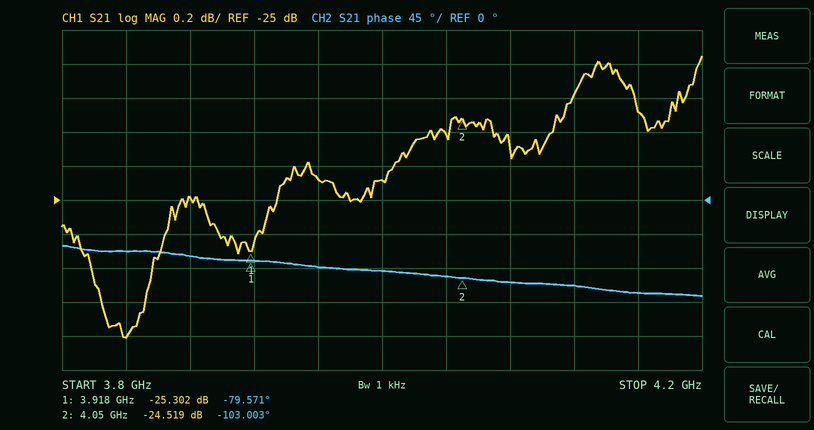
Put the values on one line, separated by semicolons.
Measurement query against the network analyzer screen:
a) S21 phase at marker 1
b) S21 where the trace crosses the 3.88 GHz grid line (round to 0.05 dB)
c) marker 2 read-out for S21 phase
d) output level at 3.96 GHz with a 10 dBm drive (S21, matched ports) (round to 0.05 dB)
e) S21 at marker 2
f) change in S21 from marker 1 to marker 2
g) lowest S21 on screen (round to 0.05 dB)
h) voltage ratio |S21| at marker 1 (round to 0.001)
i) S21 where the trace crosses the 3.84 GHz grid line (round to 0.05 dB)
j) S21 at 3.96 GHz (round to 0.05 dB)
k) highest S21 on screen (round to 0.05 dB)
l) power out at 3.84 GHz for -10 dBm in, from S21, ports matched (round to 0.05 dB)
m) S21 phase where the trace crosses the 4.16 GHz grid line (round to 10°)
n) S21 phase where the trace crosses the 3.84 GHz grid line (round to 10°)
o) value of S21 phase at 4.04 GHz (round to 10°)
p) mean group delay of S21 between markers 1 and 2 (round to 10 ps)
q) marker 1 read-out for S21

-79.571°; -25.00 dB; -103.003°; -14.90 dBm; -24.519 dB; 0.783 dB; -25.80 dB; 0.054; -25.80 dB; -24.90 dB; -24.15 dB; -35.80 dBm; -120°; -70°; -100°; 490 ps; -25.302 dB
